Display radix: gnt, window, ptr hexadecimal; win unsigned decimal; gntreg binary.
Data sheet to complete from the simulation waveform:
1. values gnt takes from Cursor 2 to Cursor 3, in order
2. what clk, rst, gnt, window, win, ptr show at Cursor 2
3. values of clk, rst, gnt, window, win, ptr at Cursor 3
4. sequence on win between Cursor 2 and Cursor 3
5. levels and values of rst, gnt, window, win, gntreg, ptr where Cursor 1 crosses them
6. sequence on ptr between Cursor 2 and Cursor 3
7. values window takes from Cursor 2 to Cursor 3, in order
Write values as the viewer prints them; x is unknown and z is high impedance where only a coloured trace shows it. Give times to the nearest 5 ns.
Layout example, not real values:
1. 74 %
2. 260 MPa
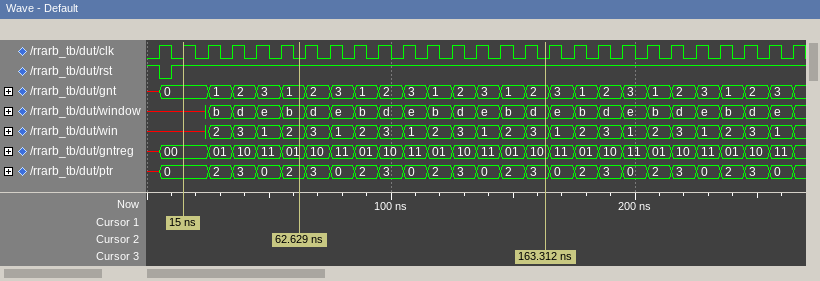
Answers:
1. 1, 2, 3, 1, 2, 3, 1, 2, 3, 1, 2
2. clk=0, rst=1, gnt=1, window=b, win=2, ptr=2
3. clk=0, rst=1, gnt=2, window=d, win=3, ptr=3
4. 2, 3, 1, 2, 3, 1, 2, 3, 1, 2, 3
5. rst=1, gnt=0, window=x, win=x, gntreg=00, ptr=0
6. 2, 3, 0, 2, 3, 0, 2, 3, 0, 2, 3
7. b, d, e, b, d, e, b, d, e, b, d
